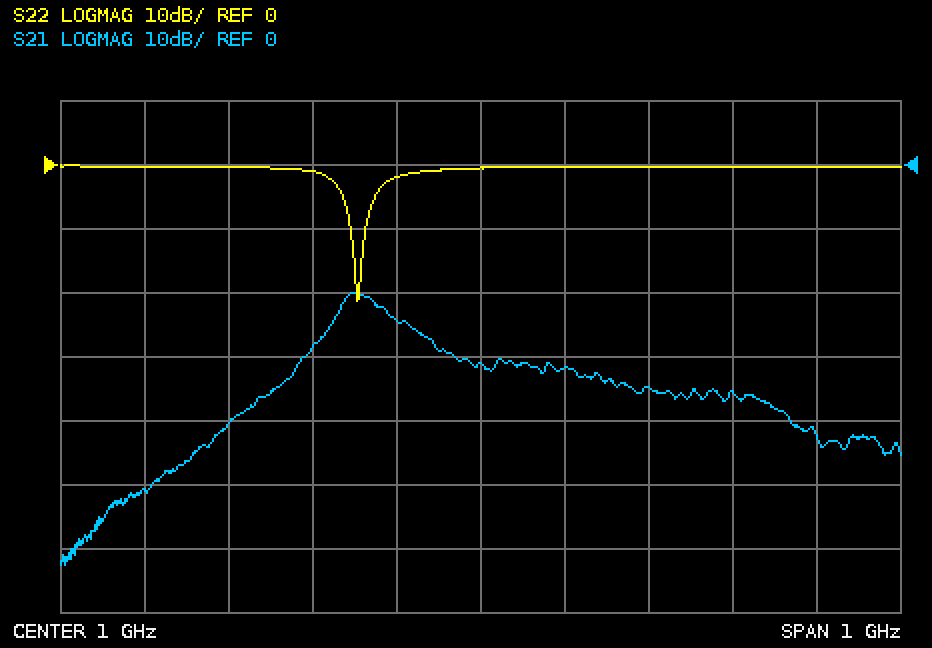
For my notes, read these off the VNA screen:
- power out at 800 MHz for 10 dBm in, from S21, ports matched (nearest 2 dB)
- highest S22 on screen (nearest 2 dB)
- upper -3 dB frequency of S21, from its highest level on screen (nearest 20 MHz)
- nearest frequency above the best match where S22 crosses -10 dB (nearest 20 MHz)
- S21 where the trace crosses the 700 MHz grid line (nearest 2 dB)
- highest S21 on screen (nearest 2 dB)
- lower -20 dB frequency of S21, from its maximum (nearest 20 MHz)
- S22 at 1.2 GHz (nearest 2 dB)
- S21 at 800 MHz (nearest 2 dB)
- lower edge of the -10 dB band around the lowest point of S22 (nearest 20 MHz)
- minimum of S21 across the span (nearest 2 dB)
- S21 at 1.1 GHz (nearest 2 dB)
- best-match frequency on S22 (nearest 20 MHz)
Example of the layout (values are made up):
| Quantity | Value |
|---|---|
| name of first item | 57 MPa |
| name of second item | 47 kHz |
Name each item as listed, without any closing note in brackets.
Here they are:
| Quantity | Value |
|---|---|
| power out at 800 MHz for 10 dBm in, from S21, ports matched | -18 dBm |
| highest S22 on screen | 0 dB |
| upper -3 dB frequency of S21, from its highest level on screen | 880 MHz |
| nearest frequency above the best match where S22 crosses -10 dB | 860 MHz |
| S21 where the trace crosses the 700 MHz grid line | -40 dB |
| highest S21 on screen | -20 dB |
| lower -20 dB frequency of S21, from its maximum | 700 MHz |
| S22 at 1.2 GHz | 0 dB |
| S21 at 800 MHz | -28 dB |
| lower edge of the -10 dB band around the lowest point of S22 | 840 MHz |
| minimum of S21 across the span | -62 dB |
| S21 at 1.1 GHz | -32 dB |
| best-match frequency on S22 | 860 MHz |
